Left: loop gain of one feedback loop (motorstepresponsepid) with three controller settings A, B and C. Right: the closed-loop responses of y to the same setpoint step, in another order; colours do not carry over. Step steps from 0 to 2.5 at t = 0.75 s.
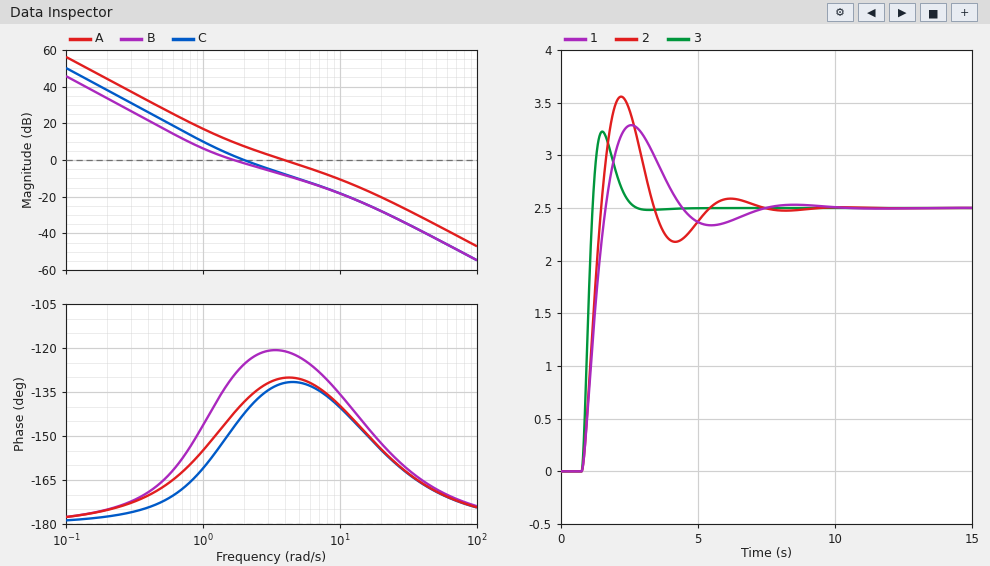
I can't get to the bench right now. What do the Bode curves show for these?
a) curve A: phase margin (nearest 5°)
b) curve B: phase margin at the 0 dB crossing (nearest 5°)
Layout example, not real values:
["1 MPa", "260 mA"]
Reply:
["50°", "50°"]
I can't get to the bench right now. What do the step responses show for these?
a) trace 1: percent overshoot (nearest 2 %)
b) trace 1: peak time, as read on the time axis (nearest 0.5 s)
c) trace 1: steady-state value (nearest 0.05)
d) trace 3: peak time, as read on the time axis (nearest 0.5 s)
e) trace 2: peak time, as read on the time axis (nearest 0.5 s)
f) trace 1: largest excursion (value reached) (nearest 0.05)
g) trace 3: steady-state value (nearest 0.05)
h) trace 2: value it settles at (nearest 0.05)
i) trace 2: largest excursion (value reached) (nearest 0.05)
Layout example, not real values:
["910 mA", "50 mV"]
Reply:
["32 %", "2.5 s", "2.50", "1.5 s", "2.0 s", "3.30", "2.50", "2.50", "3.55"]
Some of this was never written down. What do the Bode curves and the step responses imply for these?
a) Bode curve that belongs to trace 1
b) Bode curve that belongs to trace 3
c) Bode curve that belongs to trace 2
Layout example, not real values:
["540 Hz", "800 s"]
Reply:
["B", "A", "C"]
